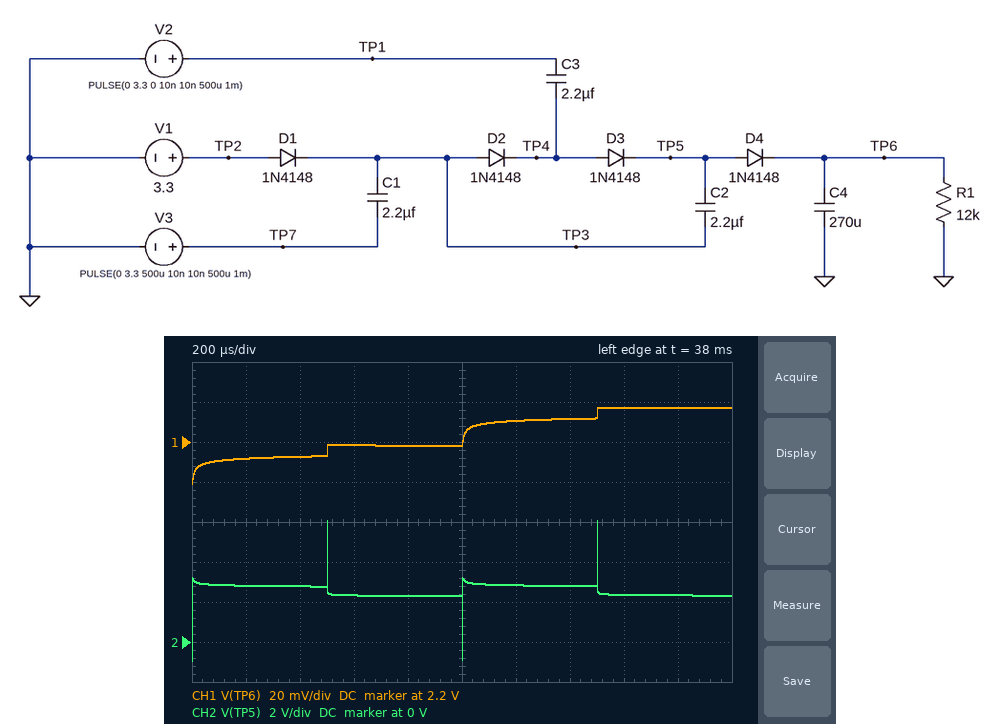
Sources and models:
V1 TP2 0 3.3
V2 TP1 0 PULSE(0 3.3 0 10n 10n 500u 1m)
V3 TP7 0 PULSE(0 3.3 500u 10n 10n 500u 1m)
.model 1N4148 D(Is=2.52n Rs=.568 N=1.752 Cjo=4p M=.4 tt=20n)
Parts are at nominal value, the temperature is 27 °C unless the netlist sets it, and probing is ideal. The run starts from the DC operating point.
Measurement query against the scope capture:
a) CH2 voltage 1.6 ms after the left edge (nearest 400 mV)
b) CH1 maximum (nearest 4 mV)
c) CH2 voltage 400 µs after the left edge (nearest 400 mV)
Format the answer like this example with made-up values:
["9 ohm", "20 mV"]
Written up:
["2.4 V", "2.216 V", "2.8 V"]
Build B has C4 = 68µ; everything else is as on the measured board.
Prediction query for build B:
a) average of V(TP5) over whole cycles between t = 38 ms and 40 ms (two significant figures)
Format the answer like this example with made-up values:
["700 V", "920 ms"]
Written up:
["4.4 V"]
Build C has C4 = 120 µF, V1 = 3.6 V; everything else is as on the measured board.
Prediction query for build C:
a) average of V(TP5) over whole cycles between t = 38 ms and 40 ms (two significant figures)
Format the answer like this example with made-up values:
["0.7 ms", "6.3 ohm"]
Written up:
["3.8 V"]
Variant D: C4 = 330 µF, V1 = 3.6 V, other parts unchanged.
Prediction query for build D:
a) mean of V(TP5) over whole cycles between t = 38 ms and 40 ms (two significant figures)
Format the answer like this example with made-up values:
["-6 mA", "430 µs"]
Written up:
["2.7 V"]
